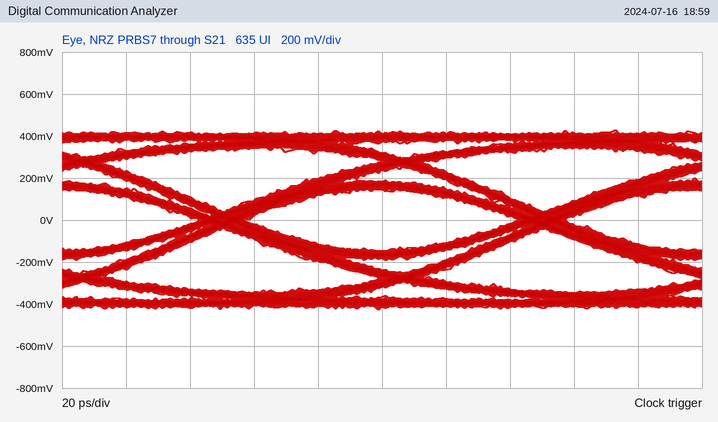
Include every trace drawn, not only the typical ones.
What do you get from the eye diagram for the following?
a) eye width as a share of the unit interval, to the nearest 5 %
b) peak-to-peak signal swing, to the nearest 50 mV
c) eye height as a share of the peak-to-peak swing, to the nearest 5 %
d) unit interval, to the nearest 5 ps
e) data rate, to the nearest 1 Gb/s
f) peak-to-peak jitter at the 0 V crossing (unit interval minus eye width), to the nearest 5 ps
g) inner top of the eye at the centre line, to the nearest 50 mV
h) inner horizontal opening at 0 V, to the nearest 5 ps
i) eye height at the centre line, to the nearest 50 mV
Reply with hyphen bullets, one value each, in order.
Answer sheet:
- 85 %
- 850 mV
- 35 %
- 100 ps
- 10 Gb/s
- 15 ps
- 150 mV
- 85 ps
- 300 mV
